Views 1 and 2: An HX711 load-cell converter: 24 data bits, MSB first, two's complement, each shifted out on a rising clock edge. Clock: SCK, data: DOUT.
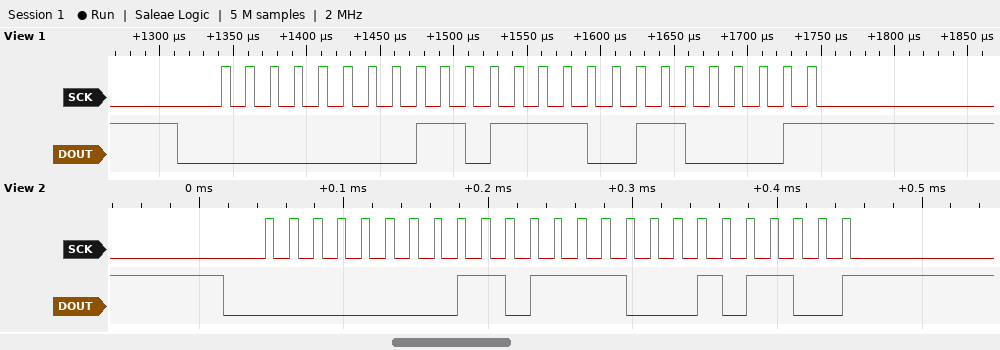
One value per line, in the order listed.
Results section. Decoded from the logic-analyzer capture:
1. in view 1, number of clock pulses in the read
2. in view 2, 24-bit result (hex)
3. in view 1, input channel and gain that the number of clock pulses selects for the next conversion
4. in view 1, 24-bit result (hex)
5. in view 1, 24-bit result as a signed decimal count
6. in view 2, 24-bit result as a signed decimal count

25
0x00DE2C
channel A, gain 128
0x00DE61
56929
56876
